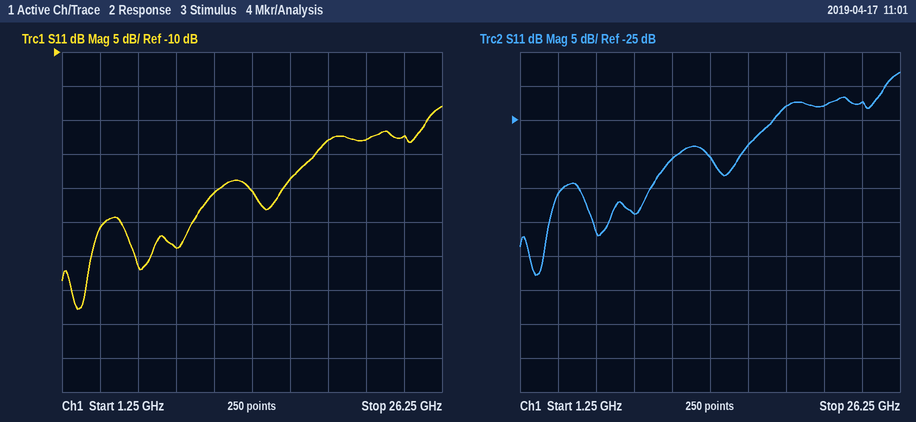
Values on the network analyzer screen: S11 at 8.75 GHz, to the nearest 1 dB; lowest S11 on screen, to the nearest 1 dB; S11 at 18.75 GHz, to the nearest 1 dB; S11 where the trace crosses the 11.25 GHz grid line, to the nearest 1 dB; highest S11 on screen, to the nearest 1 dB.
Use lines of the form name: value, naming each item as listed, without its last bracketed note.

S11 at 8.75 GHz, to the nearest 1 dB: -39 dB
lowest S11 on screen, to the nearest 1 dB: -48 dB
S11 at 18.75 GHz, to the nearest 1 dB: -23 dB
S11 where the trace crosses the 11.25 GHz grid line, to the nearest 1 dB: -31 dB
highest S11 on screen, to the nearest 1 dB: -18 dB
